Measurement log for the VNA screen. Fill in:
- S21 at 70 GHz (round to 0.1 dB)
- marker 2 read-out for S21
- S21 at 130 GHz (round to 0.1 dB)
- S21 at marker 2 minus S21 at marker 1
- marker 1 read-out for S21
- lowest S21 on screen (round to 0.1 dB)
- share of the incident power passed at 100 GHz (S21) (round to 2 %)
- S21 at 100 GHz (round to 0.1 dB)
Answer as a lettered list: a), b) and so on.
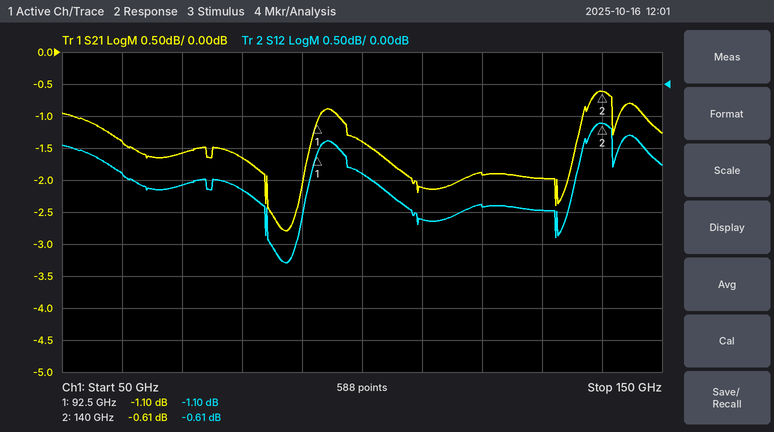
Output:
a) -1.6 dB
b) -0.61 dB
c) -2.0 dB
d) 0.49 dB
e) -1.10 dB
f) -2.8 dB
g) 72 %
h) -1.4 dB
